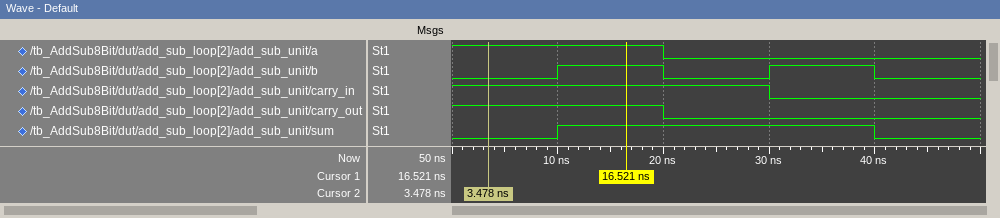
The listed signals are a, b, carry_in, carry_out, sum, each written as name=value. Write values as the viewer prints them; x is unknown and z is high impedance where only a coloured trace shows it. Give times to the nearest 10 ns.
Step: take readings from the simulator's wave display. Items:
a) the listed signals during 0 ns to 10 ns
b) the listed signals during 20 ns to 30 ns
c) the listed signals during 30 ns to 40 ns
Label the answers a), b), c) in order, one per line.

a) a=1, b=0, carry_in=1, carry_out=1, sum=0
b) a=0, b=0, carry_in=1, carry_out=0, sum=1
c) a=0, b=1, carry_in=0, carry_out=0, sum=1
